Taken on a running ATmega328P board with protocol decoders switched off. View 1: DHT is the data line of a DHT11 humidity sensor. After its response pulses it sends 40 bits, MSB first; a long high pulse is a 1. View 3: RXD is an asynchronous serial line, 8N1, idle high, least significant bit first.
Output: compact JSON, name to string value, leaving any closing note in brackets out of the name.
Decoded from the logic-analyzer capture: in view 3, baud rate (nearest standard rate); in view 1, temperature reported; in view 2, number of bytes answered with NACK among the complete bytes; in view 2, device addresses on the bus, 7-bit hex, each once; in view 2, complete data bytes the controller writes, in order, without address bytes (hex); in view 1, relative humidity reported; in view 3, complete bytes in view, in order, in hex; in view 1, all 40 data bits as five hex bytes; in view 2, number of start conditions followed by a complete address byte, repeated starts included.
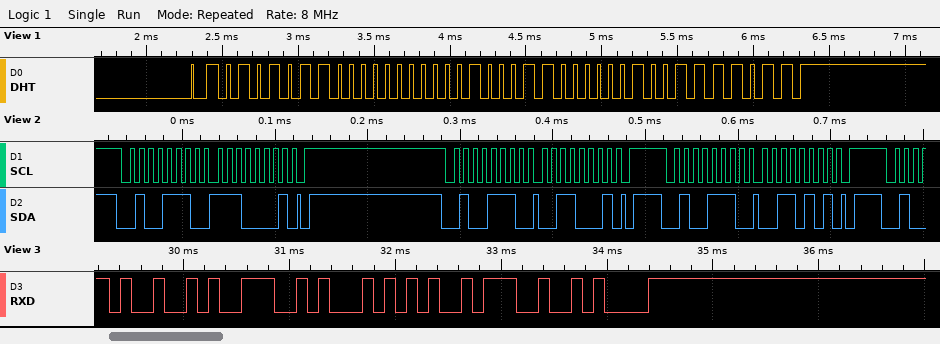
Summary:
{"in view 3, baud rate": "9600 baud", "in view 1, temperature reported": "35.2 °C", "in view 2, number of bytes answered with NACK among the complete bytes": "0", "in view 2, device addresses on the bus, 7-bit hex, each once": "0x27", "in view 2, complete data bytes the controller writes, in order, without address bytes": "E1 31 35", "in view 1, relative humidity reported": "86 %", "in view 3, complete bytes in view, in order, in hex": "49 4E 54 3A 0A", "in view 1, all 40 data bits as five hex bytes": "56 00 23 02 7B", "in view 2, number of start conditions followed by a complete address byte, repeated starts included": "3"}
